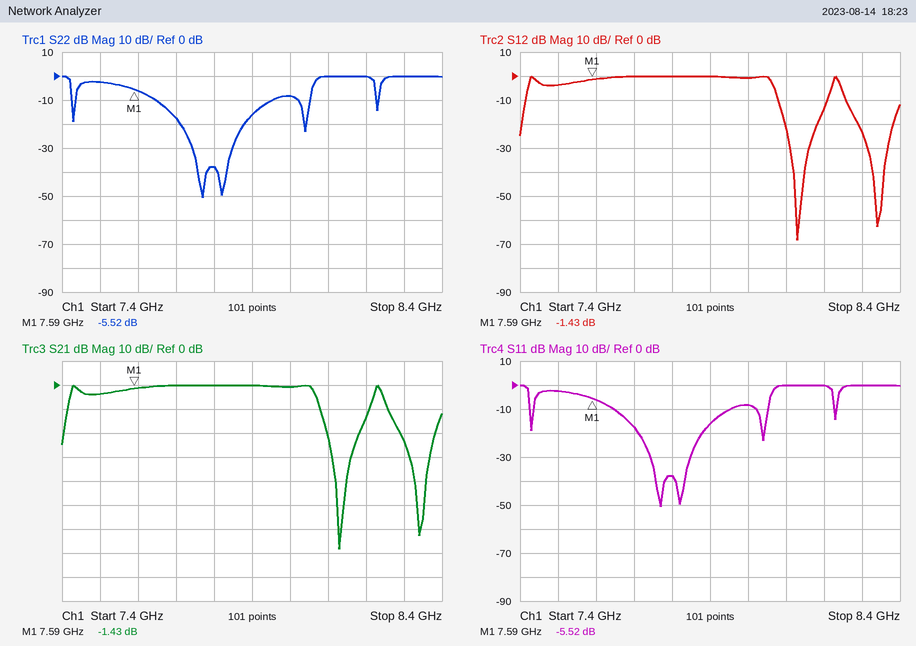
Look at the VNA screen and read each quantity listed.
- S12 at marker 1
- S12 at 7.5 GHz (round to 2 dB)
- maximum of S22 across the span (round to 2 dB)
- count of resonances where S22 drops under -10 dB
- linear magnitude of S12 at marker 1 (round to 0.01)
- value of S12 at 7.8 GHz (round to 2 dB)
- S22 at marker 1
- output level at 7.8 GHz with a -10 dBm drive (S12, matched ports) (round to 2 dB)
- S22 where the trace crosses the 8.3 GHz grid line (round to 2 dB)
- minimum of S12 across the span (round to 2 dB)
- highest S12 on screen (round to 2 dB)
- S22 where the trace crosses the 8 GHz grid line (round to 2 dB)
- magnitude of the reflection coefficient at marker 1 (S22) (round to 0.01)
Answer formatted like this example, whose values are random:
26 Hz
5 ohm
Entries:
-1.43 dB
-4 dB
0 dB
5
0.85
0 dB
-5.52 dB
-10 dBm
0 dB
-68 dB
0 dB
-8 dB
0.53
